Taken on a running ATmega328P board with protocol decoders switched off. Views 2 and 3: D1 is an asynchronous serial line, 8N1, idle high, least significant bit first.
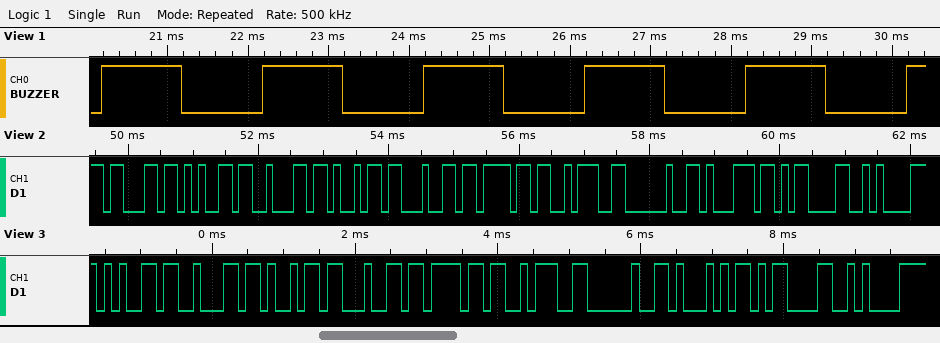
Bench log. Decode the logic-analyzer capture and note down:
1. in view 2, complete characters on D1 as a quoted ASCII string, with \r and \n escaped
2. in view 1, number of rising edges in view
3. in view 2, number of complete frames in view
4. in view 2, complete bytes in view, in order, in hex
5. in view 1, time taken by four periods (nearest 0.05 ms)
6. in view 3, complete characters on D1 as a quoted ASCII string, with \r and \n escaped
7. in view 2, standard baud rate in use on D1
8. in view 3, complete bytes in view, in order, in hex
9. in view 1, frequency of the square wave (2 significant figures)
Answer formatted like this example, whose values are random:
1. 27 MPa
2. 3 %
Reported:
1. "cebido: q\r\n"
2. 6
3. 11
4. 63 65 62 69 64 6F 3A 20 71 0D 0A
5. 8.00 ms
6. "ebido: Q\r\n"
7. 9600 baud
8. 65 62 69 64 6F 3A 20 51 0D 0A
9. 500 Hz
